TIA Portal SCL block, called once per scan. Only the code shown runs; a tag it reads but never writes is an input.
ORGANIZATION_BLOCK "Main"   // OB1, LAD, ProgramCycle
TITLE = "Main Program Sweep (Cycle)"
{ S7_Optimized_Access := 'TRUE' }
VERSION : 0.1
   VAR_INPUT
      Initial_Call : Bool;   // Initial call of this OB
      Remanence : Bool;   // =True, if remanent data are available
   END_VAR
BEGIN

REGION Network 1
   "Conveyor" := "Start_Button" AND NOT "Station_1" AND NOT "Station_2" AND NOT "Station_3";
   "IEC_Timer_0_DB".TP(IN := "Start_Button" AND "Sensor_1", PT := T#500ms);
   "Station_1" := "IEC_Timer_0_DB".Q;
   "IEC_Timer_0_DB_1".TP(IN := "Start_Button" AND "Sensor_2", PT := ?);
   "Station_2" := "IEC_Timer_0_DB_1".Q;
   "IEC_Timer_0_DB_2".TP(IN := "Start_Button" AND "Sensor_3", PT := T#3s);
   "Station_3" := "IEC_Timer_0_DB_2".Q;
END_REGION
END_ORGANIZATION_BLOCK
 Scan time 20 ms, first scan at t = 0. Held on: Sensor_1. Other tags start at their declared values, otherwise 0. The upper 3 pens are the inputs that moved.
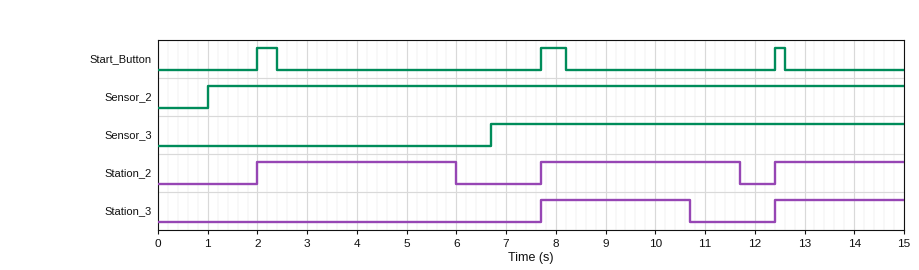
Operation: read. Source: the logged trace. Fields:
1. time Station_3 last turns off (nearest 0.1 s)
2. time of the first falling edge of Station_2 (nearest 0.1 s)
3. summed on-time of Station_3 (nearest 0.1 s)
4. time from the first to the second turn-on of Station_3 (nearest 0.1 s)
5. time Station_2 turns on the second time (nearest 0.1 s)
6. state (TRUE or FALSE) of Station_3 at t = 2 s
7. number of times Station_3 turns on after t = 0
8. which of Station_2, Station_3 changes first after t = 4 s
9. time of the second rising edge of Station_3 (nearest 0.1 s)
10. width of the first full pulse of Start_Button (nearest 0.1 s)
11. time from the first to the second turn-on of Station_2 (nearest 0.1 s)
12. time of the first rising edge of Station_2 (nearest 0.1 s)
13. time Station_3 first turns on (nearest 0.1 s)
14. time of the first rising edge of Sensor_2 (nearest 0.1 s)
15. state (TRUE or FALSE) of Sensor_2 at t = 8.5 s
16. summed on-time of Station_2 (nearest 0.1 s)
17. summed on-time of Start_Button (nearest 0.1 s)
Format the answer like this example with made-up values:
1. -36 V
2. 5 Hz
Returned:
1. 10.7 s
2. 6.0 s
3. 5.6 s
4. 4.7 s
5. 7.7 s
6. FALSE
7. 2
8. Station_2
9. 12.4 s
10. 0.4 s
11. 5.7 s
12. 2.0 s
13. 7.7 s
14. 1.0 s
15. TRUE
16. 10.6 s
17. 1.1 s
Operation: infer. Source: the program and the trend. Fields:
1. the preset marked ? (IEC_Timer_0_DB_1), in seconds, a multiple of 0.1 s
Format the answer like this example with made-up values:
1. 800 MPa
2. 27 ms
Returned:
1. 4.0 s
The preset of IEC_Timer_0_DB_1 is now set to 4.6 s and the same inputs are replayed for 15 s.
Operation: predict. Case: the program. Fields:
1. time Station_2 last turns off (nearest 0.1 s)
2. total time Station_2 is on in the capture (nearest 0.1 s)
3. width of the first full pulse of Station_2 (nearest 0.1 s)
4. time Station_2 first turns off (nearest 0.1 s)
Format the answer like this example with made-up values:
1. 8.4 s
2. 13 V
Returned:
1. 12.3 s
2. 11.8 s
3. 4.6 s
4. 6.6 s
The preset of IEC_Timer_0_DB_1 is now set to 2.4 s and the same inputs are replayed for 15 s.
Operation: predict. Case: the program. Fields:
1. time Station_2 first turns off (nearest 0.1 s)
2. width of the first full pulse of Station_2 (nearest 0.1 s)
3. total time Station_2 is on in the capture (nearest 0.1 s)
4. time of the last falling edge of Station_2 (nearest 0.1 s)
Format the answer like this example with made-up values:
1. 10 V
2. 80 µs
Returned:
1. 4.4 s
2. 2.4 s
3. 7.2 s
4. 14.8 s
